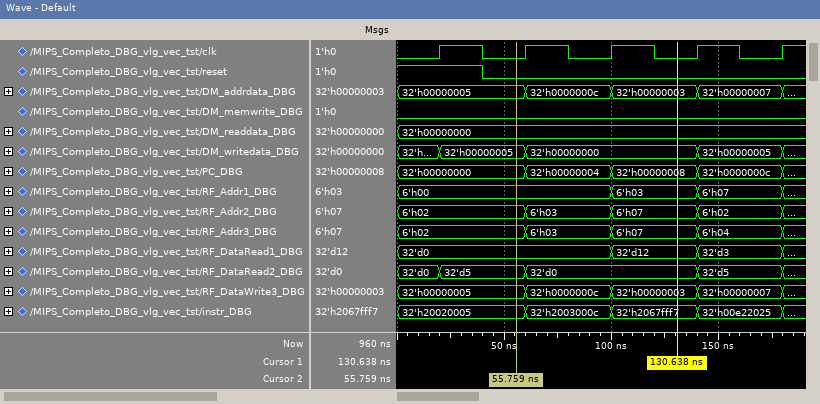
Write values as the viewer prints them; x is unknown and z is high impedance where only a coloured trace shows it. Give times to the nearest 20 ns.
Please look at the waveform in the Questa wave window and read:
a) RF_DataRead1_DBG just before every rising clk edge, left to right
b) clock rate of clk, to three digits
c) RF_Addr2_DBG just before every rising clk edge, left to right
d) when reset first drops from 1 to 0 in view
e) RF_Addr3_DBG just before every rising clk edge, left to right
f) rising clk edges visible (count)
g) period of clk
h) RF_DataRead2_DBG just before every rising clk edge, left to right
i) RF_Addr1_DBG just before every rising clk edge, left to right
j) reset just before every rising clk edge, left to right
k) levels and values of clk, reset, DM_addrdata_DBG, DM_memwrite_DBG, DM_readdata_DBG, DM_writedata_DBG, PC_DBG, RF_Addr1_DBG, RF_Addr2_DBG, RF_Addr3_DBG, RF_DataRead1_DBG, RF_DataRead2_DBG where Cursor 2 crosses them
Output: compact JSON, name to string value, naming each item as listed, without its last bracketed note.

{"RF_DataRead1_DBG just before every rising clk edge, left to right": "32'd0, 32'd0, 32'd0, 32'd12, 32'd3", "clock rate of clk, to three digits": "25.0 MHz", "RF_Addr2_DBG just before every rising clk edge, left to right": "6'h02, 6'h02, 6'h03, 6'h07, 6'h02", "when reset first drops from 1 to 0 in view": "40 ns", "RF_Addr3_DBG just before every rising clk edge, left to right": "6'h02, 6'h02, 6'h03, 6'h07, 6'h04", "rising clk edges visible": "5", "period of clk": "40 ns", "RF_DataRead2_DBG just before every rising clk edge, left to right": "32'd0, 32'd5, 32'd0, 32'd0, 32'd5", "RF_Addr1_DBG just before every rising clk edge, left to right": "6'h00, 6'h00, 6'h00, 6'h03, 6'h07", "reset just before every rising clk edge, left to right": "1 0 0 0 0", "levels and values of clk, reset, DM_addrdata_DBG, DM_memwrite_DBG, DM_readdata_DBG, DM_writedata_DBG, PC_DBG, RF_Addr1_DBG, RF_Addr2_DBG, RF_Addr3_DBG, RF_DataRead1_DBG, RF_DataRead2_DBG where Cursor 2 crosses them": "clk=0, reset=0, DM_addrdata_DBG=32'h00000005, DM_memwrite_DBG=0, DM_readdata_DBG=32'h00000000, DM_writedata_DBG=32'h00000005, PC_DBG=32'h00000000, RF_Addr1_DBG=6'h00, RF_Addr2_DBG=6'h02, RF_Addr3_DBG=6'h02, RF_DataRead1_DBG=32'd0, RF_DataRead2_DBG=32'd5"}
